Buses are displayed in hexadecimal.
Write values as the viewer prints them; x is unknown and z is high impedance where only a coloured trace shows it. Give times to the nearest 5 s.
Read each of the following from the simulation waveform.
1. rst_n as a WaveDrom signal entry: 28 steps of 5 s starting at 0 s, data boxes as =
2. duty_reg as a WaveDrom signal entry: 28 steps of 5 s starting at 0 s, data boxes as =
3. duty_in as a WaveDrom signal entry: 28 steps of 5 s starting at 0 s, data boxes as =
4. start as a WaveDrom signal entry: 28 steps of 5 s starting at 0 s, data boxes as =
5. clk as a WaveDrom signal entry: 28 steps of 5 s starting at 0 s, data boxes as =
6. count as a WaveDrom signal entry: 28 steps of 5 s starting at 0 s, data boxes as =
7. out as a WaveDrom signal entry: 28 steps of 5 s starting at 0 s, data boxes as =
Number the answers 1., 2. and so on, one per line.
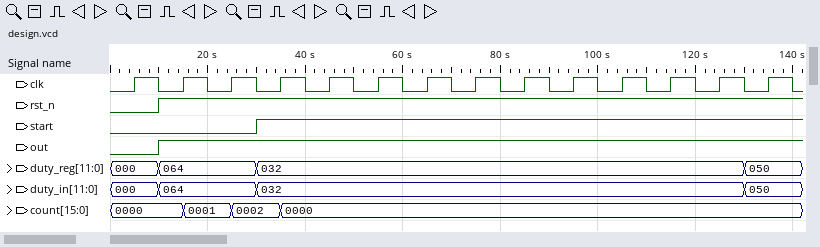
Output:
1. {name: 'rst_n', wave: '0.1.........................'}
2. {name: 'duty_reg', wave: '=.=...=...................=.', data: '000 064 032 050'}
3. {name: 'duty_in', wave: '=.=...=...................=.', data: '000 064 032 050'}
4. {name: 'start', wave: '0.....1.....................'}
5. {name: 'clk', wave: '0101010101010101010101010101'}
6. {name: 'count', wave: '=..=.=.=....................', data: '0000 0001 0002 0000'}
7. {name: 'out', wave: '0.1.........................'}
